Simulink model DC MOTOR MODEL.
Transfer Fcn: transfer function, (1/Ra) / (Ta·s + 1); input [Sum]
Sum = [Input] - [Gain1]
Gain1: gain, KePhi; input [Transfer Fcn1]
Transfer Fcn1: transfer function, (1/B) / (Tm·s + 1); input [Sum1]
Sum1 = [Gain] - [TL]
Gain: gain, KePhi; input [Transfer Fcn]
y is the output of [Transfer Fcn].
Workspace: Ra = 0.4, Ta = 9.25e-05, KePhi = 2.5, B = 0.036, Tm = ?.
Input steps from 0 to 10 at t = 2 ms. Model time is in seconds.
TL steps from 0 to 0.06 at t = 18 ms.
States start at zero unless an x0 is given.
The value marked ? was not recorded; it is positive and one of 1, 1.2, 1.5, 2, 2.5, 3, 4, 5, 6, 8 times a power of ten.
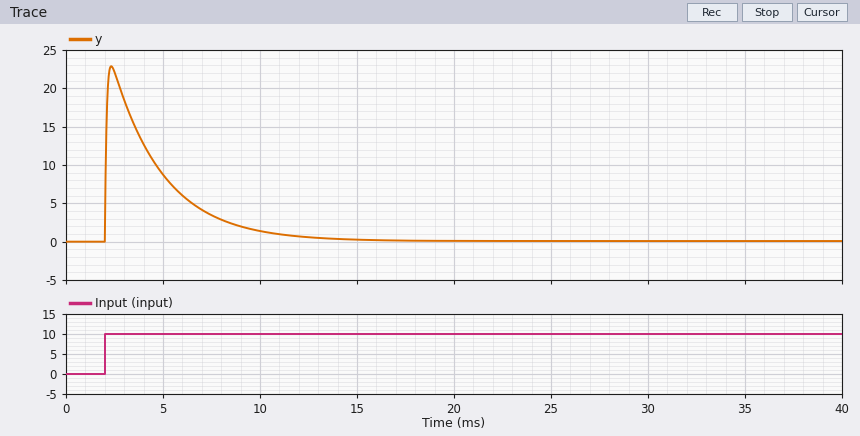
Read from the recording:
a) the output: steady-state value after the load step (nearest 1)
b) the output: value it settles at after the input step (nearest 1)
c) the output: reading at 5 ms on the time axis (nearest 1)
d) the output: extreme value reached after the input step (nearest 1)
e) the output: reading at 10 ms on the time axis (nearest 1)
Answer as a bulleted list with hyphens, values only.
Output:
- 0
- 0
- 9
- 23
- 1
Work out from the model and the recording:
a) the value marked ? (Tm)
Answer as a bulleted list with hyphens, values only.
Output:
- 1.2
